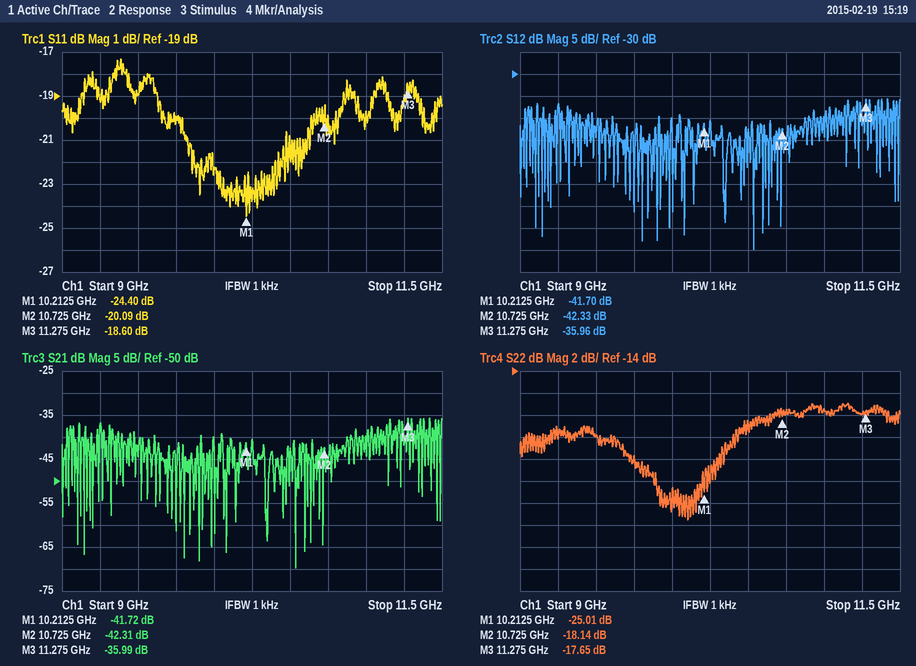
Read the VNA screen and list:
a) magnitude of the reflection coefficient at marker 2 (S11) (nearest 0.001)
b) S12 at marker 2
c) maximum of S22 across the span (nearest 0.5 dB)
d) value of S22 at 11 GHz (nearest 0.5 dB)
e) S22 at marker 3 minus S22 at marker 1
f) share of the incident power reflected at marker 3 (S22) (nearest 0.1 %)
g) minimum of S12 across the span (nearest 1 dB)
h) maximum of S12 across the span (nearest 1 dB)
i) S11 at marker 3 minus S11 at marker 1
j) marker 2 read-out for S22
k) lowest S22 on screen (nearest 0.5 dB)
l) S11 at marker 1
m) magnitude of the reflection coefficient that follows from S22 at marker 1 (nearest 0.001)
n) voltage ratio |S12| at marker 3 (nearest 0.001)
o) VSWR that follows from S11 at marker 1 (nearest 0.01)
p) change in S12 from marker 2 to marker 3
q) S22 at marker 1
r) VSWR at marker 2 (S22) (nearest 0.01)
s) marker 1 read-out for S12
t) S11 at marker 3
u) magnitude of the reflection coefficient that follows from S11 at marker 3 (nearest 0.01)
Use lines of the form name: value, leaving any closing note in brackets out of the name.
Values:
magnitude of the reflection coefficient at marker 2 (S11): 0.099
S12 at marker 2: -42.33 dB
maximum of S22 across the span: -17.0 dB
value of S22 at 11 GHz: -17.5 dB
S22 at marker 3 minus S22 at marker 1: 7.36 dB
share of the incident power reflected at marker 3 (S22): 1.7 %
minimum of S12 across the span: -70 dB
maximum of S12 across the span: -36 dB
S11 at marker 3 minus S11 at marker 1: 5.80 dB
marker 2 read-out for S22: -18.14 dB
lowest S22 on screen: -27.5 dB
S11 at marker 1: -24.40 dB
magnitude of the reflection coefficient that follows from S22 at marker 1: 0.056
voltage ratio |S12| at marker 3: 0.016
VSWR that follows from S11 at marker 1: 1.13
change in S12 from marker 2 to marker 3: 6.37 dB
S22 at marker 1: -25.01 dB
VSWR at marker 2 (S22): 1.28
marker 1 read-out for S12: -41.70 dB
S11 at marker 3: -18.60 dB
magnitude of the reflection coefficient that follows from S11 at marker 3: 0.12
